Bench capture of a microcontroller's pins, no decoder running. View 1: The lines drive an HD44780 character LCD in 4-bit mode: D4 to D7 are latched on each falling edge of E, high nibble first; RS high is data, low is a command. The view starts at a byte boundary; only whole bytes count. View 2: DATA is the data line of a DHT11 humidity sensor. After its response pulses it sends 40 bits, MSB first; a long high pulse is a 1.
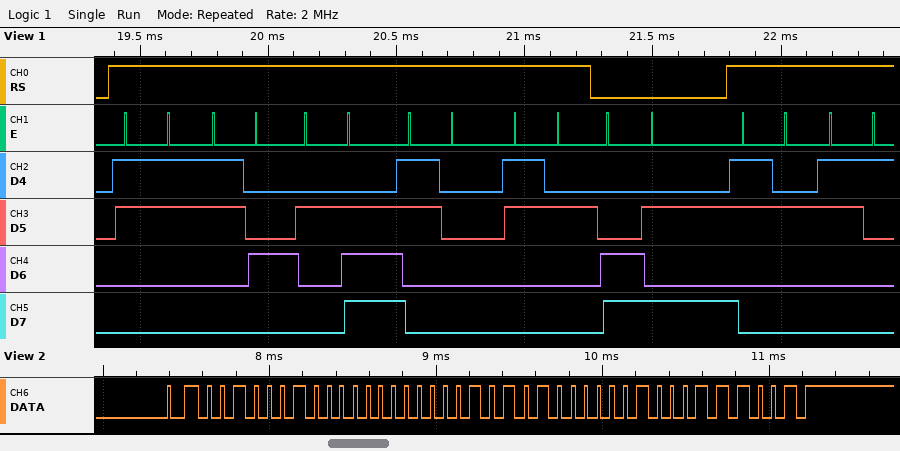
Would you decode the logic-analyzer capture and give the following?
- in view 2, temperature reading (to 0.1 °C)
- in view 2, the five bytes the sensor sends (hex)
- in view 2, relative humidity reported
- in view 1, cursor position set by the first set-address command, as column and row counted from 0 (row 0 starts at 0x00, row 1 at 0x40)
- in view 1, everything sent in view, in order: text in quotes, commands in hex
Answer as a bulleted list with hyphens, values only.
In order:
- 21.2 °C
- 22 00 15 02 39
- 34 %
- column 10, row 1
- "34.02" 0xCA "21"
